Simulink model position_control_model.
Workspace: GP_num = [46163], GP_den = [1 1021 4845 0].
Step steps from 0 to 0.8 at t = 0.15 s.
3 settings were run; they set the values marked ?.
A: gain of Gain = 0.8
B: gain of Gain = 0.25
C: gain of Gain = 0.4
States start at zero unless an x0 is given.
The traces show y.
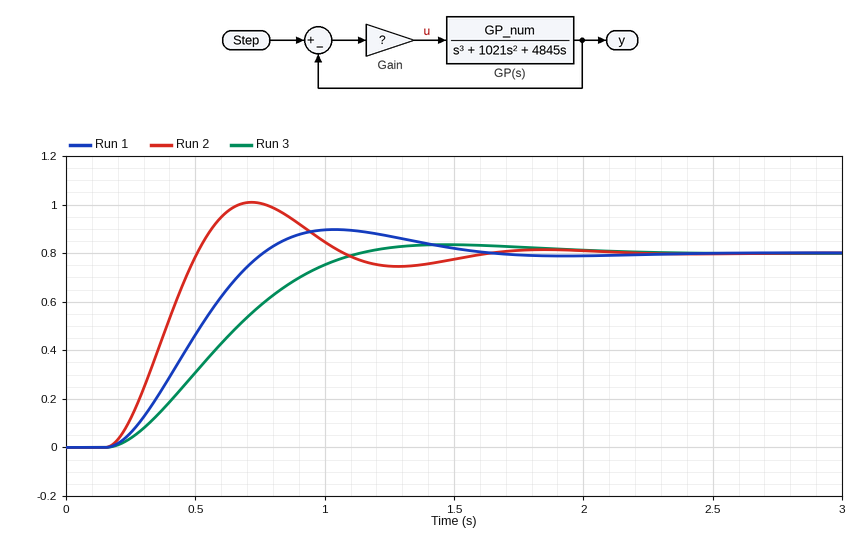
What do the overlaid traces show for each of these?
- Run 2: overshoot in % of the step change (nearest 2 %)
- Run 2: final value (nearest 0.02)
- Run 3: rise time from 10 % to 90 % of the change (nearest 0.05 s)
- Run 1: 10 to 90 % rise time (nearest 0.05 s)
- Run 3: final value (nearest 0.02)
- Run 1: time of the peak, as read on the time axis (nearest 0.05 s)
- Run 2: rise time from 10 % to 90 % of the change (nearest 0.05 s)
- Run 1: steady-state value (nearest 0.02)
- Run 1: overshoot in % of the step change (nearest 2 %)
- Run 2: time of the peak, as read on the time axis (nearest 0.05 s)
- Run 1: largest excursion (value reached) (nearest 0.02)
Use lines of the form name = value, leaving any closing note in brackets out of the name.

Run 2: overshoot in % of the step change = 26 %
Run 2: final value = 0.80
Run 3: rise time from 10 % to 90 % of the change = 0.65 s
Run 1: 10 to 90 % rise time = 0.40 s
Run 3: final value = 0.80
Run 1: time of the peak, as read on the time axis = 1.05 s
Run 2: rise time from 10 % to 90 % of the change = 0.25 s
Run 1: steady-state value = 0.80
Run 1: overshoot in % of the step change = 12 %
Run 2: time of the peak, as read on the time axis = 0.70 s
Run 1: largest excursion (value reached) = 0.90
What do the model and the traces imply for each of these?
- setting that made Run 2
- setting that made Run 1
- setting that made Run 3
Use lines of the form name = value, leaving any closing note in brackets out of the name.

setting that made Run 2 = A
setting that made Run 1 = C
setting that made Run 3 = B
